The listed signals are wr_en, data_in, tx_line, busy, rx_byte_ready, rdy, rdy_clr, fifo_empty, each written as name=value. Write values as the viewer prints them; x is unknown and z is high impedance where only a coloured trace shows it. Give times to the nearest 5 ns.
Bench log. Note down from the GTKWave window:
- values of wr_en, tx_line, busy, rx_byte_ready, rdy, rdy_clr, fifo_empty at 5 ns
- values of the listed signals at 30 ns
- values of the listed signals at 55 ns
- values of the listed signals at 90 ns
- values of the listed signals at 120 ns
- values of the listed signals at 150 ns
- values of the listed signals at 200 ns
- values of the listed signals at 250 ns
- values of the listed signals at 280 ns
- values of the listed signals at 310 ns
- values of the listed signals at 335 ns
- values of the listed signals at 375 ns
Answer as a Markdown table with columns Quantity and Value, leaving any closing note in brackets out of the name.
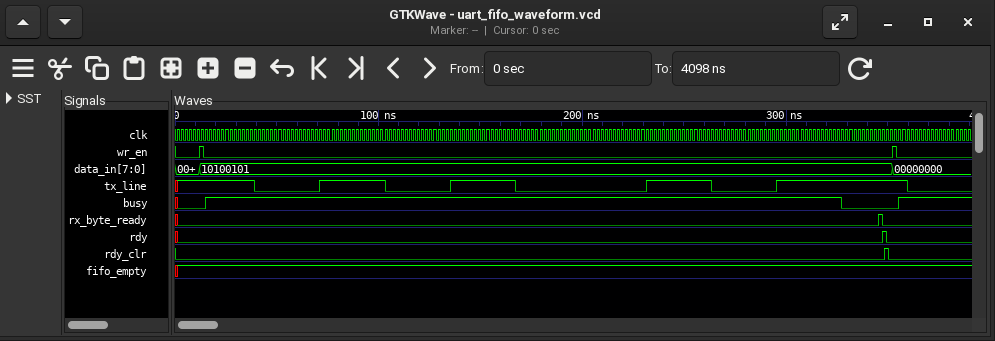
| Quantity | Value |
|---|---|
| values of wr_en, tx_line, busy, rx_byte_ready, rdy, rdy_clr, fifo_empty at 5 ns | wr_en=0, tx_line=1, busy=0, rx_byte_ready=0, rdy=0, rdy_clr=0, fifo_empty=1 |
| values of the listed signals at 30 ns | wr_en=0, data_in=10100101, tx_line=1, busy=1, rx_byte_ready=0, rdy=0, rdy_clr=0, fifo_empty=1 |
| values of the listed signals at 55 ns | wr_en=0, data_in=10100101, tx_line=0, busy=1, rx_byte_ready=0, rdy=0, rdy_clr=0, fifo_empty=1 |
| values of the listed signals at 90 ns | wr_en=0, data_in=10100101, tx_line=1, busy=1, rx_byte_ready=0, rdy=0, rdy_clr=0, fifo_empty=1 |
| values of the listed signals at 120 ns | wr_en=0, data_in=10100101, tx_line=0, busy=1, rx_byte_ready=0, rdy=0, rdy_clr=0, fifo_empty=1 |
| values of the listed signals at 150 ns | wr_en=0, data_in=10100101, tx_line=1, busy=1, rx_byte_ready=0, rdy=0, rdy_clr=0, fifo_empty=1 |
| values of the listed signals at 200 ns | wr_en=0, data_in=10100101, tx_line=0, busy=1, rx_byte_ready=0, rdy=0, rdy_clr=0, fifo_empty=1 |
| values of the listed signals at 250 ns | wr_en=0, data_in=10100101, tx_line=1, busy=1, rx_byte_ready=0, rdy=0, rdy_clr=0, fifo_empty=1 |
| values of the listed signals at 280 ns | wr_en=0, data_in=10100101, tx_line=0, busy=1, rx_byte_ready=0, rdy=0, rdy_clr=0, fifo_empty=1 |
| values of the listed signals at 310 ns | wr_en=0, data_in=10100101, tx_line=1, busy=1, rx_byte_ready=0, rdy=0, rdy_clr=0, fifo_empty=1 |
| values of the listed signals at 335 ns | wr_en=0, data_in=10100101, tx_line=1, busy=0, rx_byte_ready=0, rdy=0, rdy_clr=0, fifo_empty=1 |
| values of the listed signals at 375 ns | wr_en=0, data_in=00000000, tx_line=0, busy=1, rx_byte_ready=0, rdy=0, rdy_clr=0, fifo_empty=1 |
